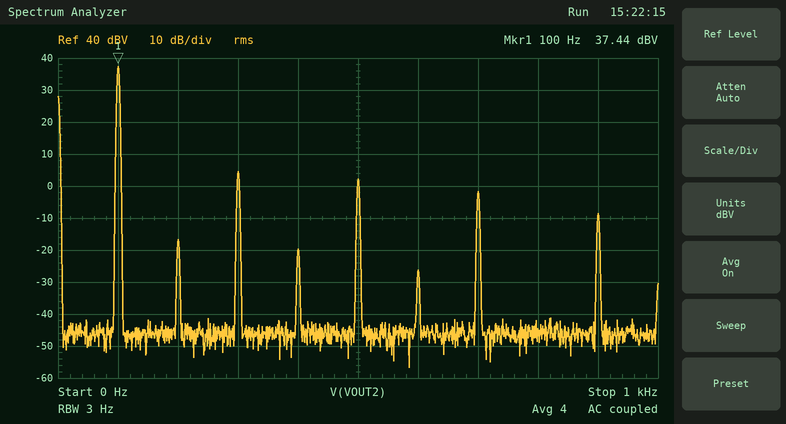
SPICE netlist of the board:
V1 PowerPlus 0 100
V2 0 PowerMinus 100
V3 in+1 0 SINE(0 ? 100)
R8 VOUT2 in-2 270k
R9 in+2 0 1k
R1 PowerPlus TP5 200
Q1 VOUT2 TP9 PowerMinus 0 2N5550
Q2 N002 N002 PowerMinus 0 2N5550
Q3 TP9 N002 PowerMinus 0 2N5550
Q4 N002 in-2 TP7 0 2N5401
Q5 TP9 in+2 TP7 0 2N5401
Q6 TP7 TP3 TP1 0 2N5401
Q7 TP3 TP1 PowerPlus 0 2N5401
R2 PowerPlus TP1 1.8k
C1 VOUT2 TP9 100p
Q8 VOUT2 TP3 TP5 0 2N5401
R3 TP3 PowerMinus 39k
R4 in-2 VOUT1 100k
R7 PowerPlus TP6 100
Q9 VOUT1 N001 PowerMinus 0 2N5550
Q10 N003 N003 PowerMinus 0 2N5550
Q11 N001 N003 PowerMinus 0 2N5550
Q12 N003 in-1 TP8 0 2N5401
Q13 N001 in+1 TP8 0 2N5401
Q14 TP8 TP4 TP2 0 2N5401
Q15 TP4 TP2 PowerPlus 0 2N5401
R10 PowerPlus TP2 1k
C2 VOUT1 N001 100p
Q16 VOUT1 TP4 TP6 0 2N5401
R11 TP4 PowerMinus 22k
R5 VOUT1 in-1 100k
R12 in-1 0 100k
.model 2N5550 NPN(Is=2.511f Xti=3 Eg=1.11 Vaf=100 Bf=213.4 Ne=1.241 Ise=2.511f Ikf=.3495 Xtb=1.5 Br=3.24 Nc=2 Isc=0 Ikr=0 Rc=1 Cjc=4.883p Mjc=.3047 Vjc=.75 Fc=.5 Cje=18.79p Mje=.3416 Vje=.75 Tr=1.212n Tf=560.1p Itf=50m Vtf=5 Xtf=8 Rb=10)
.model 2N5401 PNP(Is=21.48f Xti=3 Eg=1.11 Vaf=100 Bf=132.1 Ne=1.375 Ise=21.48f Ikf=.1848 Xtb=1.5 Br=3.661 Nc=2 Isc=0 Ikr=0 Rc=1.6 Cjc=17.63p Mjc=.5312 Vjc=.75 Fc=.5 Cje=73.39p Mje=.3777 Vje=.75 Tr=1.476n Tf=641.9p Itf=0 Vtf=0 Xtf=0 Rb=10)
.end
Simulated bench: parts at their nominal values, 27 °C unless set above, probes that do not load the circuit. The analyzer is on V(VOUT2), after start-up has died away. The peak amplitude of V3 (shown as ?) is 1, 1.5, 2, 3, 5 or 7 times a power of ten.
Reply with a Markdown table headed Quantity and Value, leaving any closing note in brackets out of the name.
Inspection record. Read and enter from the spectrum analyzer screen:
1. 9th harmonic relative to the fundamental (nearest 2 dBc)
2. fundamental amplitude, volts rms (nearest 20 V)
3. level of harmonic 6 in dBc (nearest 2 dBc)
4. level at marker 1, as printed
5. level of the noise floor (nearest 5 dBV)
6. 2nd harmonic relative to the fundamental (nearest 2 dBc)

| Quantity | Value |
|---|---|
| 9th harmonic relative to the fundamental | -46 dBc |
| fundamental amplitude, volts rms | 80 V |
| level of harmonic 6 in dBc | -64 dBc |
| level at marker 1, as printed | 37.44 dBV |
| level of the noise floor | -45 dBV |
| 2nd harmonic relative to the fundamental | -54 dBc |
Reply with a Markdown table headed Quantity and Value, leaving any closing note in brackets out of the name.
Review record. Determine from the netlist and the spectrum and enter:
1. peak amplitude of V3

| Quantity | Value |
|---|---|
| peak amplitude of V3 | 20 V |
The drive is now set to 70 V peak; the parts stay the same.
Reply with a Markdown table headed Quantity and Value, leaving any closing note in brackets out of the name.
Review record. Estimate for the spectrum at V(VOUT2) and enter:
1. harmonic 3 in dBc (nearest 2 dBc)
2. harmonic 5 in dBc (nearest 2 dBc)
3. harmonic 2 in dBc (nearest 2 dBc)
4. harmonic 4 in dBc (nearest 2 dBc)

| Quantity | Value |
|---|---|
| harmonic 3 in dBc | -10 dBc |
| harmonic 5 in dBc | -16 dBc |
| harmonic 2 in dBc | -58 dBc |
| harmonic 4 in dBc | -60 dBc |
